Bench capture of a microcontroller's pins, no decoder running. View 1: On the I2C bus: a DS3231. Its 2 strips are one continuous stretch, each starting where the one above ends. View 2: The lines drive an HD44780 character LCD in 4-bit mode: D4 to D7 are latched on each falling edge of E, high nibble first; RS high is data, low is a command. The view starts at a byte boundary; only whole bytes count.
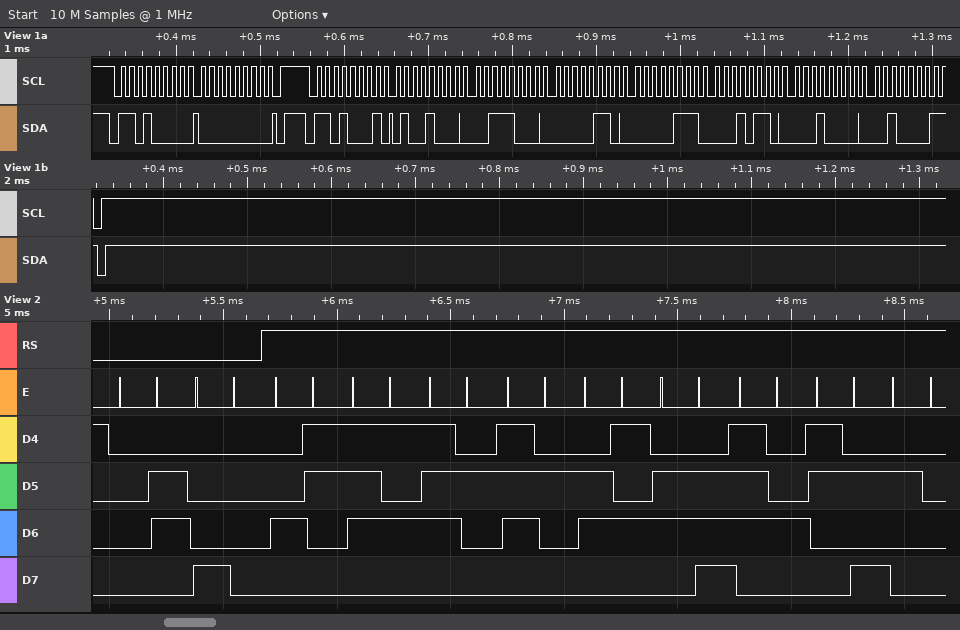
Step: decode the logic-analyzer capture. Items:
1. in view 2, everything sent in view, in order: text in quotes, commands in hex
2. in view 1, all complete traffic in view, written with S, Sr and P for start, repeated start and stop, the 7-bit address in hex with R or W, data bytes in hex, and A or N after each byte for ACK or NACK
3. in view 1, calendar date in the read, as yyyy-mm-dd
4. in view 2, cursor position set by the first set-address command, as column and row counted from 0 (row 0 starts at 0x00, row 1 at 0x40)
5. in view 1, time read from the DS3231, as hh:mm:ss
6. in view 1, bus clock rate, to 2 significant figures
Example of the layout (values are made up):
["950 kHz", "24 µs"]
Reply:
["0x06 0x80 \"Current: \"", "S 68W A 00 A P S 68R A 48 A 38 A 06 A 07 A 16 A 10 A 21 N P", "2021-10-16", "column 0, row 0", "06:38:48", "100 kHz"]
